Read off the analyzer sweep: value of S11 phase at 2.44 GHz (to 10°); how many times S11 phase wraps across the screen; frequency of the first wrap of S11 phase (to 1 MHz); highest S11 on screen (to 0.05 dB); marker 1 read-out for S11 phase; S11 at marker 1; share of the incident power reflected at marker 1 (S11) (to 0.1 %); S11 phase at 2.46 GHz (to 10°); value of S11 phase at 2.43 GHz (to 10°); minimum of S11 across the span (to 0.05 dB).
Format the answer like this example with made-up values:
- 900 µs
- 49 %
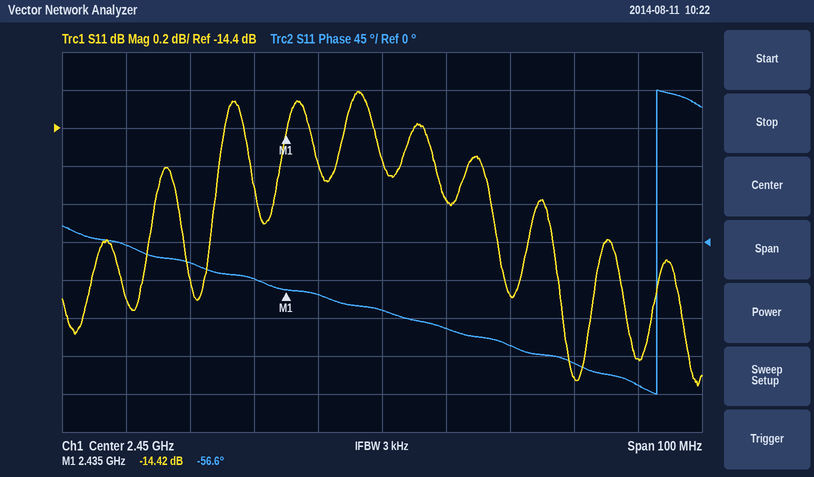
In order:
- -60°
- 1
- 2.493 GHz
- -14.20 dB
- -56.6°
- -14.42 dB
- 3.6 %
- -100°
- -40°
- -15.75 dB
